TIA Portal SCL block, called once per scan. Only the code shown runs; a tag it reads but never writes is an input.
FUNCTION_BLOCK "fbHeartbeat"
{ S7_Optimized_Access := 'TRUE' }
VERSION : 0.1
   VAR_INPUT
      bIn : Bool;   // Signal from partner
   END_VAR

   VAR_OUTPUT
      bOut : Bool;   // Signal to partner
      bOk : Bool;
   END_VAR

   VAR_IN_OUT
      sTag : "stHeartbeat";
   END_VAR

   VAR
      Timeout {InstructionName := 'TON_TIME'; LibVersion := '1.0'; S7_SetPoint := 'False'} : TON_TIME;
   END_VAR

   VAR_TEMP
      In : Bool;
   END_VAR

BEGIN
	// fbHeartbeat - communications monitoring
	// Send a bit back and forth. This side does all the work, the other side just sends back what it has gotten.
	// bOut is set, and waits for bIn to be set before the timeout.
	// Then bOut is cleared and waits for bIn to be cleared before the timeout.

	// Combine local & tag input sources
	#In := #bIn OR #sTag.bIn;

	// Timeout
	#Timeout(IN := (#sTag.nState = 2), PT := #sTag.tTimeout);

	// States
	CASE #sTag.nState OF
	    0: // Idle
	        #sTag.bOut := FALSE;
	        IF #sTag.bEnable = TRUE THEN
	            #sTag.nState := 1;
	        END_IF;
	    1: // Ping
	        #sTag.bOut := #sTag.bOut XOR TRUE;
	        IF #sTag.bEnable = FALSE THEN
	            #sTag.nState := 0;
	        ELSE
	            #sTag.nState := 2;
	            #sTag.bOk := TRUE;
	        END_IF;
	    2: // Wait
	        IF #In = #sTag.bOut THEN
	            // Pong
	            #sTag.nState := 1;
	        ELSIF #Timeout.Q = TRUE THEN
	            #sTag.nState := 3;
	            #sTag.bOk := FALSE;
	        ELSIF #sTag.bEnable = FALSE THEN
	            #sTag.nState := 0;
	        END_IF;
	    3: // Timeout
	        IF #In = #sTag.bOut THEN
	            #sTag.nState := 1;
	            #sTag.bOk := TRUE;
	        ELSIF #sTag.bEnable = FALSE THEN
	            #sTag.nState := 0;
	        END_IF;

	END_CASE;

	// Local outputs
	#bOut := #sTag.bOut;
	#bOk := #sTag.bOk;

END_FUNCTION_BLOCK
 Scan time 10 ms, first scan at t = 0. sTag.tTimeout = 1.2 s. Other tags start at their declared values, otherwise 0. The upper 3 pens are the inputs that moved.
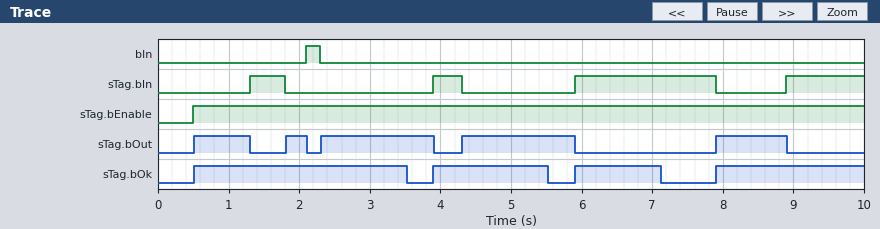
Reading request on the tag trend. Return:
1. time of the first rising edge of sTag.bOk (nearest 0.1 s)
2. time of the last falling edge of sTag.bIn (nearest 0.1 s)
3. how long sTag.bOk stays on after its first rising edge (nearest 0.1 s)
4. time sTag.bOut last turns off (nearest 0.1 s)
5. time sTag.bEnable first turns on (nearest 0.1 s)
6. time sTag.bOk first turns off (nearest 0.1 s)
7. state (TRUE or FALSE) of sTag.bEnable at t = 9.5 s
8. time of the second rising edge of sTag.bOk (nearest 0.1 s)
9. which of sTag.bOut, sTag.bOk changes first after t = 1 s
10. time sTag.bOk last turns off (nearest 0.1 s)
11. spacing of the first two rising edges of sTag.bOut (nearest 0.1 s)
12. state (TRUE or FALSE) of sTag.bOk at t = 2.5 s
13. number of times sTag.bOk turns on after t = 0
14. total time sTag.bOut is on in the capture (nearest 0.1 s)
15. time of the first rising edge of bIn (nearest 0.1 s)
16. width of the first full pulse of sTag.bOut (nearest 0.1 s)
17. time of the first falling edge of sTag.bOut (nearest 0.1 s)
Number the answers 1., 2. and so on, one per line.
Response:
1. 0.5 s
2. 7.9 s
3. 3.0 s
4. 8.9 s
5. 0.5 s
6. 3.5 s
7. TRUE
8. 3.9 s
9. sTag.bOut
10. 7.1 s
11. 1.3 s
12. TRUE
13. 4
14. 5.3 s
15. 2.1 s
16. 0.8 s
17. 1.3 s
